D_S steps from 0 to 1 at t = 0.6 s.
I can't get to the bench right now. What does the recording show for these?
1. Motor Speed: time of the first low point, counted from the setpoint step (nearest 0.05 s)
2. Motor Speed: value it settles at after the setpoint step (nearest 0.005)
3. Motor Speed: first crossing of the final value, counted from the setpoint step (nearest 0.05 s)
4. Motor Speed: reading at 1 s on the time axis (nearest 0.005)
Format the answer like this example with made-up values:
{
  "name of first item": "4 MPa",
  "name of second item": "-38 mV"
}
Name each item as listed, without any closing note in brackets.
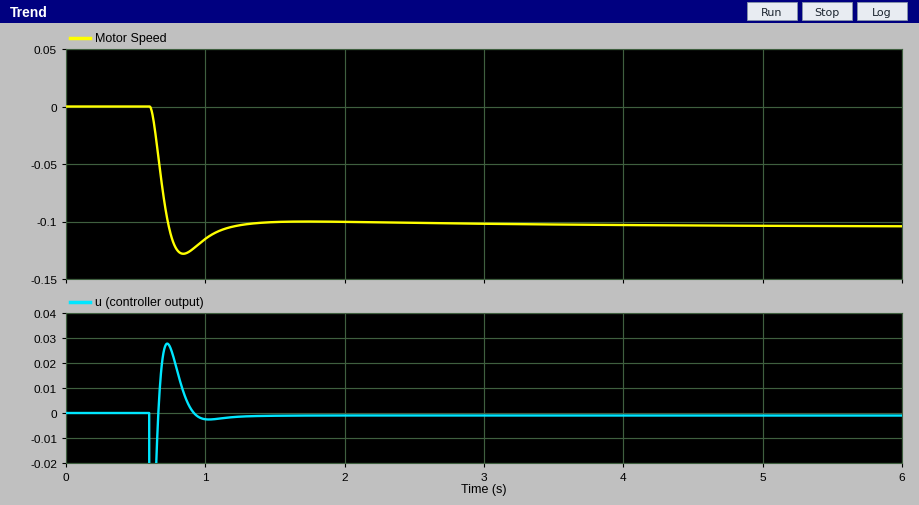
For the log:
{
  "Motor Speed: time of the first low point, counted from the setpoint step": "0.25 s",
  "Motor Speed: value it settles at after the setpoint step": "-0.105",
  "Motor Speed: first crossing of the final value, counted from the setpoint step": "0.15 s",
  "Motor Speed: reading at 1 s on the time axis": "-0.115"
}
